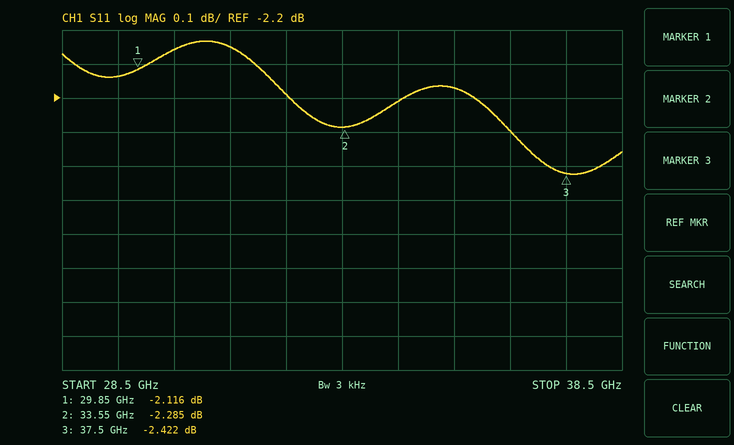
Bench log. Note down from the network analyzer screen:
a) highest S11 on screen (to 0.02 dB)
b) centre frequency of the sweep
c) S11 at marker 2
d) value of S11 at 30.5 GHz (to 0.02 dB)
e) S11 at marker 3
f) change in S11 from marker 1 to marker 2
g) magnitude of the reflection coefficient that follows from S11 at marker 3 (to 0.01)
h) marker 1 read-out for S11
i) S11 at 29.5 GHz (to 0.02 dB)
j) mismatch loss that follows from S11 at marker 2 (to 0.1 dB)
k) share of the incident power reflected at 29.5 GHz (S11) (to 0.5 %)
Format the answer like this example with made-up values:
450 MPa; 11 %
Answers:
-2.04 dB; 33.5 GHz; -2.285 dB; -2.06 dB; -2.422 dB; -0.169 dB; 0.76; -2.116 dB; -2.14 dB; 3.9 dB; 61.0 %
